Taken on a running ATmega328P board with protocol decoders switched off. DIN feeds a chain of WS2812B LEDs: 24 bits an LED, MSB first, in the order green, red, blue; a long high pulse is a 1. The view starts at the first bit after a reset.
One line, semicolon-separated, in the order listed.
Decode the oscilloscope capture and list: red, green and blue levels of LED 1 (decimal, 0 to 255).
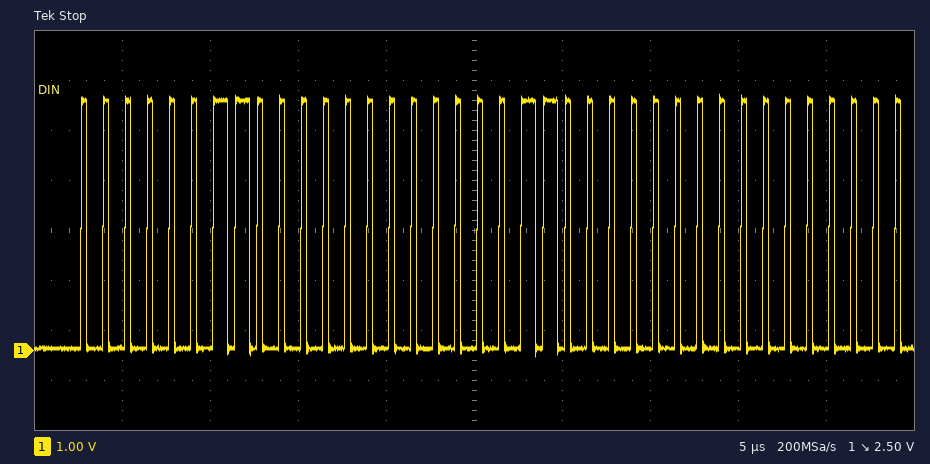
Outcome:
0, 3, 12
